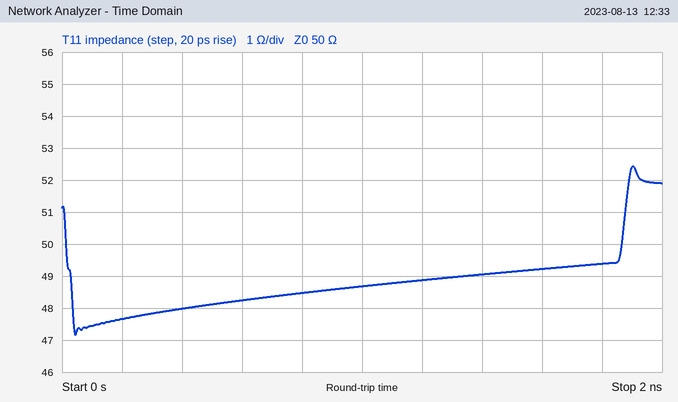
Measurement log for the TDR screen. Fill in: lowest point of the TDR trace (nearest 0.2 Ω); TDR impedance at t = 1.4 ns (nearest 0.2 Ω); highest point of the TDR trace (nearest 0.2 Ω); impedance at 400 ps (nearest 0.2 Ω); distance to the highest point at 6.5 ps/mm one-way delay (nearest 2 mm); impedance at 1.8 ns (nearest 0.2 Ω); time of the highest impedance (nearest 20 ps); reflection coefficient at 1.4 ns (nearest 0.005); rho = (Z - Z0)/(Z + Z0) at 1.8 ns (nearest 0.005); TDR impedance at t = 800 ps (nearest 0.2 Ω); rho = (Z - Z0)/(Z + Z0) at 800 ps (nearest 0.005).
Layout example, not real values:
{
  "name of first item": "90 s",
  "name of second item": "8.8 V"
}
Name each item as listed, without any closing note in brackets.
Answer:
{
  "lowest point of the TDR trace": "47.2 Ω",
  "TDR impedance at t = 1.4 ns": "49.0 Ω",
  "highest point of the TDR trace": "52.4 Ω",
  "impedance at 400 ps": "48.0 Ω",
  "distance to the highest point at 6.5 ps/mm one-way delay": "146 mm",
  "impedance at 1.8 ns": "49.4 Ω",
  "time of the highest impedance": "1.90 ns",
  "reflection coefficient at 1.4 ns": "-0.010",
  "rho = (Z - Z0)/(Z + Z0) at 1.8 ns": "-0.005",
  "TDR impedance at t = 800 ps": "48.4 Ω",
  "rho = (Z - Z0)/(Z + Z0) at 800 ps": "-0.015"
}
